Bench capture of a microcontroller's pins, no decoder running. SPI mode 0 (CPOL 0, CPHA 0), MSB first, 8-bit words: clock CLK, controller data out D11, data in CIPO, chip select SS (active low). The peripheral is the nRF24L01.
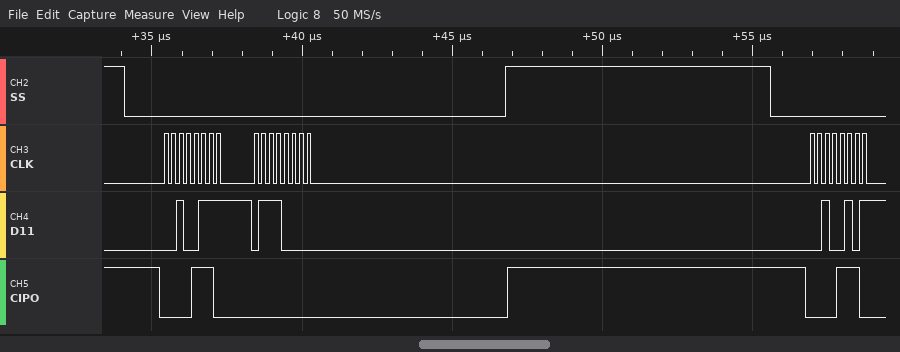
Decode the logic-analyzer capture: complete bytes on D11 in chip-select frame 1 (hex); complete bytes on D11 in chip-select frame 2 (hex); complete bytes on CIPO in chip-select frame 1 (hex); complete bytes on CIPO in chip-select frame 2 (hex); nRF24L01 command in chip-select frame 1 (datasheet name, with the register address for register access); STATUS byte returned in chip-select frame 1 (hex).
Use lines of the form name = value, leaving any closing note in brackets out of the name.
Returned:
complete bytes on D11 in chip-select frame 1 = 27 70
complete bytes on D11 in chip-select frame 2 = 25
complete bytes on CIPO in chip-select frame 1 = 0E 00
complete bytes on CIPO in chip-select frame 2 = 0E
nRF24L01 command in chip-select frame 1 = W_REGISTER 0x07
STATUS byte returned in chip-select frame 1 = 0x0E
